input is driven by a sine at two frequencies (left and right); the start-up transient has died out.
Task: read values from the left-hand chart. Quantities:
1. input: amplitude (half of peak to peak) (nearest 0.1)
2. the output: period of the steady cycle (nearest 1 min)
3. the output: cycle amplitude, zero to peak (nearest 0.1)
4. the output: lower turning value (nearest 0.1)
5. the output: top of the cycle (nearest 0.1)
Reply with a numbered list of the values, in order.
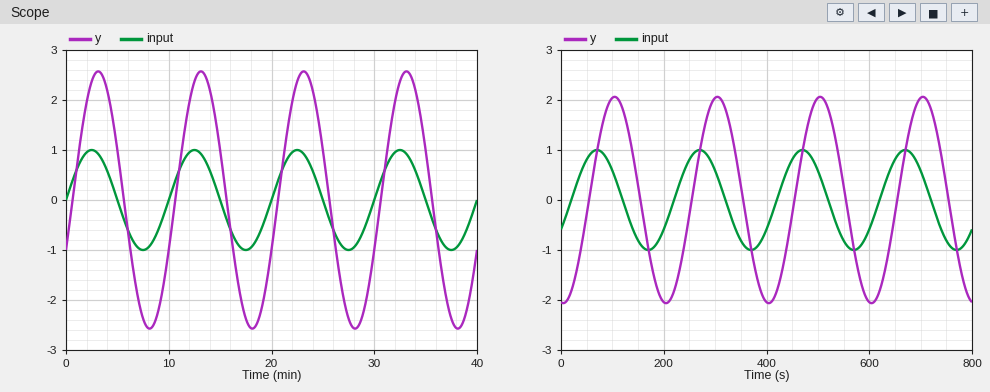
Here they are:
1. 1.0
2. 10 min
3. 2.6
4. -2.6
5. 2.6
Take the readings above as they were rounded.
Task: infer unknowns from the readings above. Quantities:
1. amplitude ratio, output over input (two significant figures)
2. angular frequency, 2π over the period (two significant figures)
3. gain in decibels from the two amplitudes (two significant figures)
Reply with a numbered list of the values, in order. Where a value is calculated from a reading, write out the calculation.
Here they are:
1. 2.6 / 1 = 2.6
2. 2π / 10 = 0.63 rad/min
3. 20 log10(2.6 / 1) = 8.3 dB
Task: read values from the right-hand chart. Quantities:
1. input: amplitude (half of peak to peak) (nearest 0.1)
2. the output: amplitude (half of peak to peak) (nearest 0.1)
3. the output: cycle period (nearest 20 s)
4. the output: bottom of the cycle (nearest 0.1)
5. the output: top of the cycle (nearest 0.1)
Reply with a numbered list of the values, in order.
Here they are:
1. 1.0
2. 2.1
3. 200 s
4. -2.1
5. 2.1
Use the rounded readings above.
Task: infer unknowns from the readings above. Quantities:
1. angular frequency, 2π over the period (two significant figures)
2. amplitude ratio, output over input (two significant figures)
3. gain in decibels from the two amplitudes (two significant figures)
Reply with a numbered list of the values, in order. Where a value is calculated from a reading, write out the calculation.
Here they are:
1. 2π / 200 = 0.031 rad/s
2. 2.1 / 1 = 2.1
3. 20 log10(2.1 / 1) = 6.4 dB
